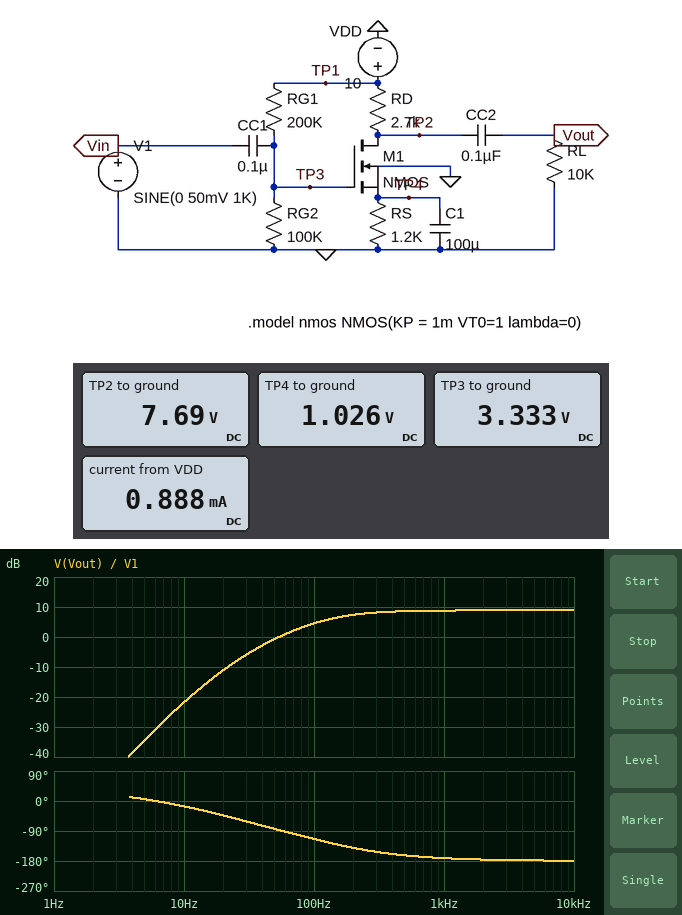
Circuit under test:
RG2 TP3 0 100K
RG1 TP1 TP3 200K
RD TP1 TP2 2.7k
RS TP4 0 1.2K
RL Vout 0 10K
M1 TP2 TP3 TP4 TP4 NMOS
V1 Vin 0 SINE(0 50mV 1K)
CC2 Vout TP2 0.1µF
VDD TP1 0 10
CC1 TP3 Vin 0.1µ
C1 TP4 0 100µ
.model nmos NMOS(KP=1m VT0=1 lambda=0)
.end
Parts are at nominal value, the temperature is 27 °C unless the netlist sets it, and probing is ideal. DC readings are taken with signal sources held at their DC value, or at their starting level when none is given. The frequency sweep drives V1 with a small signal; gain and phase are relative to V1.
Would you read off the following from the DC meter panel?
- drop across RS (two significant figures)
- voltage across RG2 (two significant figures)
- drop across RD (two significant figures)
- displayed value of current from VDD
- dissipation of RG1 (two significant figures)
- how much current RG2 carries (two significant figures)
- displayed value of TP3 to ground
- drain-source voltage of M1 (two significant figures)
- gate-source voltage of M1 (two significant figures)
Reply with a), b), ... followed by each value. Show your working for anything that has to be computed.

a) 1.026 V = 1.0 V
b) 3.333 V = 3.3 V
c) 10 V - 7.69 V = 2.3 V
d) 0.888 mA
e) (10 V - 3.333 V)^2 / 200 kΩ = 220 µW
f) (3.333 V) / 100 kΩ = 33 µA
g) 3.333 V
h) 7.69 V - 1.026 V = 6.7 V
i) 3.333 V - 1.026 V = 2.3 V
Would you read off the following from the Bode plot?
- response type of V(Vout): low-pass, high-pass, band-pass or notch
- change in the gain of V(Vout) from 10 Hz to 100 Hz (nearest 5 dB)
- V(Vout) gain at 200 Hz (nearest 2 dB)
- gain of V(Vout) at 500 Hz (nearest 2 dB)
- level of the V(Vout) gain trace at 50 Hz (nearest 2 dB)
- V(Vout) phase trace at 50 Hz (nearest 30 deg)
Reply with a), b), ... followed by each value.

a) high-pass
b) 25 dB
c) 8 dB
d) 8 dB
e) 0 dB
f) -90 deg
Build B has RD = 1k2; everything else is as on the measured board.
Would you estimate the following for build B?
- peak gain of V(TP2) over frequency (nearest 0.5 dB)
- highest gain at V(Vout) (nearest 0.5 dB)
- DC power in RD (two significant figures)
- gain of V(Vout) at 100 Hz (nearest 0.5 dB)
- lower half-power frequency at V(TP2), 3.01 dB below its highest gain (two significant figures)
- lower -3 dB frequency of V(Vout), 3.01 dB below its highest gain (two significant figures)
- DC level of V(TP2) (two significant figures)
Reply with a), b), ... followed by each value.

a) 3.5 dB
b) 3.0 dB
c) 880 µW
d) -2.0 dB
e) 22 Hz
f) 150 Hz
g) 9.0 V
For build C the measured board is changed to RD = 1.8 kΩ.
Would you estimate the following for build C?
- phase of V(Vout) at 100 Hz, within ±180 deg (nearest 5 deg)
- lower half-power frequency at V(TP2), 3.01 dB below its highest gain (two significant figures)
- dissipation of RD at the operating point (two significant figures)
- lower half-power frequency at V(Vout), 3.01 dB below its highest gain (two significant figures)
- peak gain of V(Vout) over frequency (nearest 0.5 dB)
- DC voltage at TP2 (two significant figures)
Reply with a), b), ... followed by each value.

a) -110 deg
b) 21 Hz
c) 1.3 mW
d) 140 Hz
e) 6.0 dB
f) 8.5 V
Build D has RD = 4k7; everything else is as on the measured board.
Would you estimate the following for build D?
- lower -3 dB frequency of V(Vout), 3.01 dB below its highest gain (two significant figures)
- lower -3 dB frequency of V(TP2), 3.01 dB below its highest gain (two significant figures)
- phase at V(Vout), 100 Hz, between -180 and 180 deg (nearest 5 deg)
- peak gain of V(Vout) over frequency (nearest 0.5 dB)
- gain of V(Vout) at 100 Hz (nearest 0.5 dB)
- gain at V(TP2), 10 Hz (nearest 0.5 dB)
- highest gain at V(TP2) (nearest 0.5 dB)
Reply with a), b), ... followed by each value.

a) 110 Hz
b) 19 Hz
c) -120 deg
d) 12.5 dB
e) 9.0 dB
f) 7.0 dB
g) 14.5 dB
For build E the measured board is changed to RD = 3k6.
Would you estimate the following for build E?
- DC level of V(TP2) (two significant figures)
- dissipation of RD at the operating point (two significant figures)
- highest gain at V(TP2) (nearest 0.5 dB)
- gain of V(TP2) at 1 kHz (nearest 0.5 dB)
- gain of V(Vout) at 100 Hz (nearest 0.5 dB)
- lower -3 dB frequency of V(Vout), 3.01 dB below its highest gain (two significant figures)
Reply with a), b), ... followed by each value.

a) 6.9 V
b) 2.6 mW
c) 12.5 dB
d) 11.0 dB
e) 7.0 dB
f) 120 Hz
